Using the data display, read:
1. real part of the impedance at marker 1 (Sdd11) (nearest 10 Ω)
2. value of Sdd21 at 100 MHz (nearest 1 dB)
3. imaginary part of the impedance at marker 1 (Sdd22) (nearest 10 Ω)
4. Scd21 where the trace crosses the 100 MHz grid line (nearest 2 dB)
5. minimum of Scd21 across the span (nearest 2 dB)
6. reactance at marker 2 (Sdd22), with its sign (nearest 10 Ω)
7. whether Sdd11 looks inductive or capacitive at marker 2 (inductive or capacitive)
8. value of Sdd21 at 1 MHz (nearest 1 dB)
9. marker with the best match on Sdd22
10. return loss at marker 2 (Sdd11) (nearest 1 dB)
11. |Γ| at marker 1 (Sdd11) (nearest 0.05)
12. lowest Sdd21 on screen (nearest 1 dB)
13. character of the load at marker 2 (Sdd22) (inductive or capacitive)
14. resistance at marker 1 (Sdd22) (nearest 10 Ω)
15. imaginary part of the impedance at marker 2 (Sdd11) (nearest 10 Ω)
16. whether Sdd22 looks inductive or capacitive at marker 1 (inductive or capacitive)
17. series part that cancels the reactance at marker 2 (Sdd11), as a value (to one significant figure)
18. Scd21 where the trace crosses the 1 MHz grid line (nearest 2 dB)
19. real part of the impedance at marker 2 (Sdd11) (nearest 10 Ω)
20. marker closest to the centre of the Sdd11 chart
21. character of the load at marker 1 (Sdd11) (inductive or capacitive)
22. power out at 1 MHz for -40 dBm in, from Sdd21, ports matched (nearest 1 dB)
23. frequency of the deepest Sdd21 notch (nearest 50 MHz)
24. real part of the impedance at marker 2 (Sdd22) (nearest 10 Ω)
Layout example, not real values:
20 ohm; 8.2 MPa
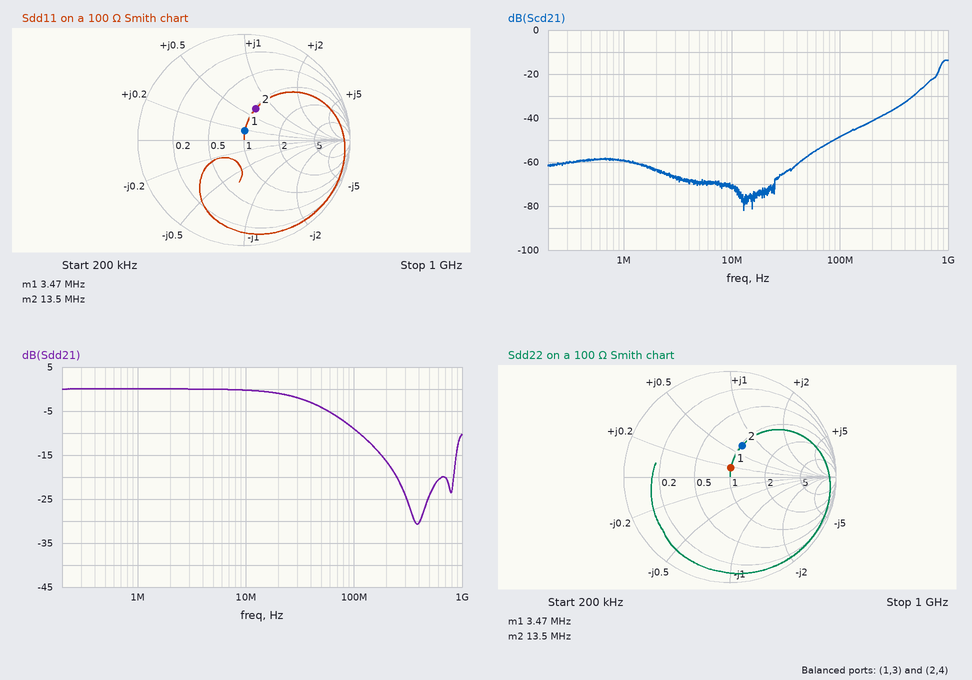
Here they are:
100 Ω; -9 dB; +20 Ω; -48 dB; -82 dB; +70 Ω; inductive; 0 dB; marker 1; 10 dB; 0.10; -31 dB; inductive; 100 Ω; +70 Ω; inductive; 200 pF; -60 dB; 100 Ω; marker 1; inductive; -40 dBm; 400 MHz; 100 Ω
